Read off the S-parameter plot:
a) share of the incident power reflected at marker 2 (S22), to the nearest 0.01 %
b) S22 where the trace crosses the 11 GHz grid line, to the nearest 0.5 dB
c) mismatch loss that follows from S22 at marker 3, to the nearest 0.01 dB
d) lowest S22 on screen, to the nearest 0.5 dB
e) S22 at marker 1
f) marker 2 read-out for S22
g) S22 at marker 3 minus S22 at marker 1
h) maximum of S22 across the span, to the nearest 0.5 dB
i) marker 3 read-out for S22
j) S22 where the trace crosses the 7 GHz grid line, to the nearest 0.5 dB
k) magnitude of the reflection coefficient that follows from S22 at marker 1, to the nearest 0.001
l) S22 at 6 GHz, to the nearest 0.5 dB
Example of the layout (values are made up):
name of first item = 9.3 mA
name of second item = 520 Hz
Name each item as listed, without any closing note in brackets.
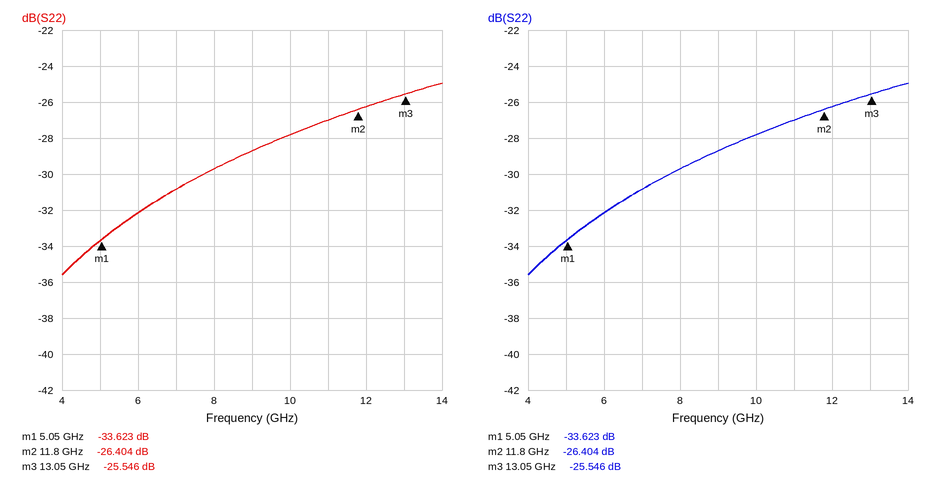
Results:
share of the incident power reflected at marker 2 (S22), to the nearest 0.01 % = 0.23 %
S22 where the trace crosses the 11 GHz grid line, to the nearest 0.5 dB = -27.0 dB
mismatch loss that follows from S22 at marker 3, to the nearest 0.01 dB = 0.01 dB
lowest S22 on screen, to the nearest 0.5 dB = -35.5 dB
S22 at marker 1 = -33.623 dB
marker 2 read-out for S22 = -26.404 dB
S22 at marker 3 minus S22 at marker 1 = 8.077 dB
maximum of S22 across the span, to the nearest 0.5 dB = -25.0 dB
marker 3 read-out for S22 = -25.546 dB
S22 where the trace crosses the 7 GHz grid line, to the nearest 0.5 dB = -31.0 dB
magnitude of the reflection coefficient that follows from S22 at marker 1, to the nearest 0.001 = 0.021
S22 at 6 GHz, to the nearest 0.5 dB = -32.0 dB
